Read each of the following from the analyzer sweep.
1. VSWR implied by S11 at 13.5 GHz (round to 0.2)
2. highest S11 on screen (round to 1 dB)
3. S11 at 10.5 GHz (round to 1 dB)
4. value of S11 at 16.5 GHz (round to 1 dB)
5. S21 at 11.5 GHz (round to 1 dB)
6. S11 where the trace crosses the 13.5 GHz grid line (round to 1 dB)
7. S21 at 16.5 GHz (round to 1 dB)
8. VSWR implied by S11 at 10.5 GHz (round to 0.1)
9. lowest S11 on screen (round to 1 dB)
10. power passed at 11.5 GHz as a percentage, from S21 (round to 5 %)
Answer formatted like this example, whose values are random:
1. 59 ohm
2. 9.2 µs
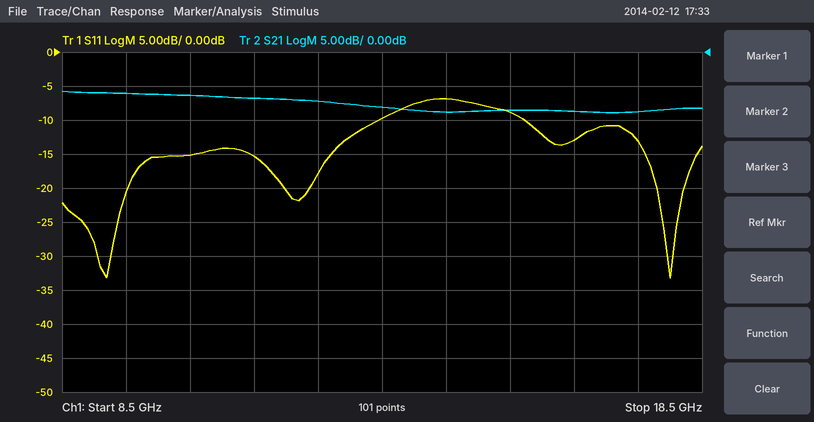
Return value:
1. 2.0
2. -7 dB
3. -15 dB
4. -13 dB
5. -7 dB
6. -10 dB
7. -9 dB
8. 1.4
9. -33 dB
10. 20 %
